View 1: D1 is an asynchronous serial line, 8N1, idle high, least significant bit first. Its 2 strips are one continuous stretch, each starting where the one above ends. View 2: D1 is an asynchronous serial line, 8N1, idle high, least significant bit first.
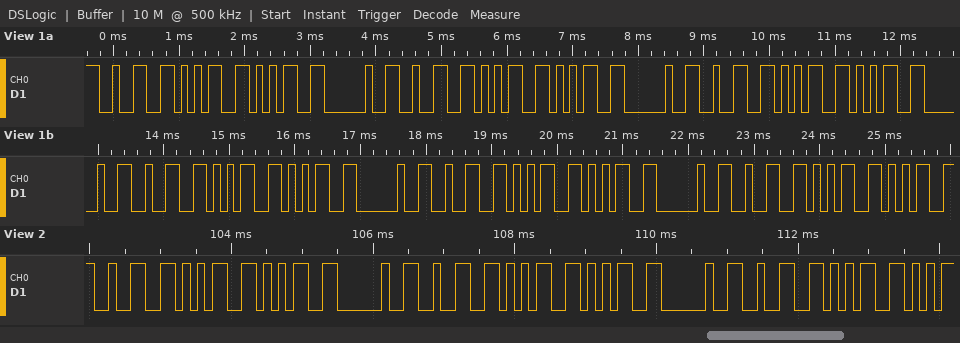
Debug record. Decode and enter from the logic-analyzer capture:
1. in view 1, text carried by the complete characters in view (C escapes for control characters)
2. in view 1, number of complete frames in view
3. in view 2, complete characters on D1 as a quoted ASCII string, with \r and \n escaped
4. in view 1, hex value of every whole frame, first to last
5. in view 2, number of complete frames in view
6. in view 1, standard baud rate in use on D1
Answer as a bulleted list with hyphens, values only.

- "255 255 255 255 255 255"
- 23
- "255 255 25"
- 32 35 35 20 32 35 35 20 32 35 35 20 32 35 35 20 32 35 35 20 32 35 35
- 10
- 9600 baud
